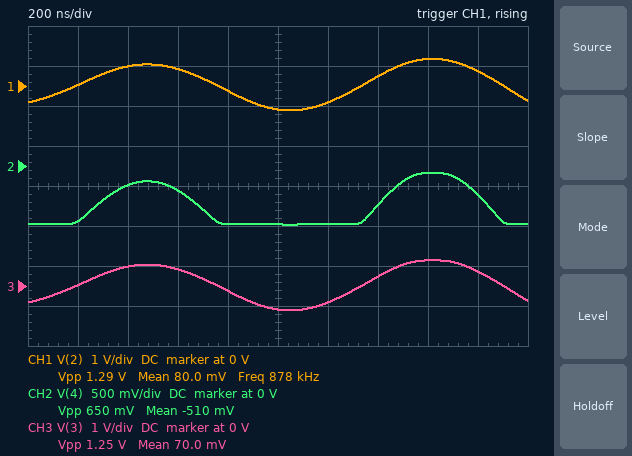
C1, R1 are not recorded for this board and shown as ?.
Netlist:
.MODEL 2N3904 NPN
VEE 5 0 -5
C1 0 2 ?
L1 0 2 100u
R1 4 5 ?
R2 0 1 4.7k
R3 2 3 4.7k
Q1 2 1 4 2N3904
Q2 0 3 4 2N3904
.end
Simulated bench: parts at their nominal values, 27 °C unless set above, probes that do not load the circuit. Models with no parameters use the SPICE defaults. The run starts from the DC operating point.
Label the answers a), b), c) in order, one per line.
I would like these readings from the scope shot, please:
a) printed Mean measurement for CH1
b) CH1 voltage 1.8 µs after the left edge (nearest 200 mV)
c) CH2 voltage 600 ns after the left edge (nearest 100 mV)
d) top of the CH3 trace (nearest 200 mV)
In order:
a) 80.0 mV
b) 400 mV
c) -300 mV
d) 600 mV
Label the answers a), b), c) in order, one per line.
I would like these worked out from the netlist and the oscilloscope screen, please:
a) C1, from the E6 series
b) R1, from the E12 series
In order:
a) 330 pF
b) 33 kΩ
